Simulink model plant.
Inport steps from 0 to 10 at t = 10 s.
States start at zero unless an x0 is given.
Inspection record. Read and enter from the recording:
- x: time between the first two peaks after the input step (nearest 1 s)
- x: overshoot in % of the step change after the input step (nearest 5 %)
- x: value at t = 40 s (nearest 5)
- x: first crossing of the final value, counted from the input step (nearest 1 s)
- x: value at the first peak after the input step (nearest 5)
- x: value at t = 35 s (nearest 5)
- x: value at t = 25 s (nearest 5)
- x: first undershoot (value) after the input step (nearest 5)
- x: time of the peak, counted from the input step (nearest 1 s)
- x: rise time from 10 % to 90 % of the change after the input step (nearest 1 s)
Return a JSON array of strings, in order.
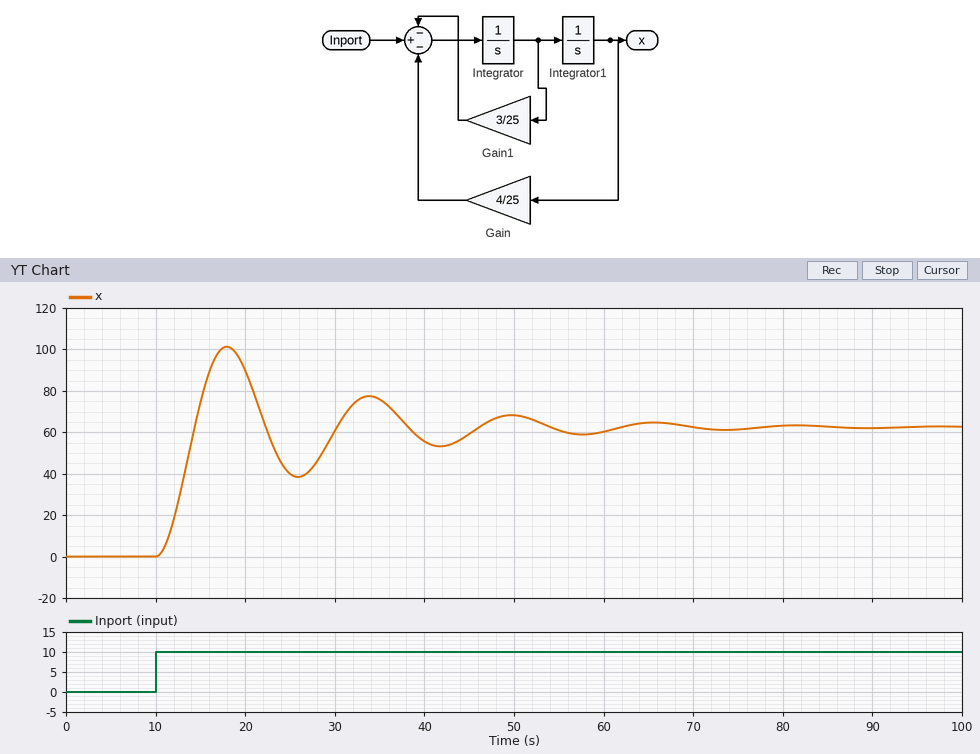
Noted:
["16 s", "60 %", "55", "4 s", "100", "75", "40", "40", "8 s", "3 s"]
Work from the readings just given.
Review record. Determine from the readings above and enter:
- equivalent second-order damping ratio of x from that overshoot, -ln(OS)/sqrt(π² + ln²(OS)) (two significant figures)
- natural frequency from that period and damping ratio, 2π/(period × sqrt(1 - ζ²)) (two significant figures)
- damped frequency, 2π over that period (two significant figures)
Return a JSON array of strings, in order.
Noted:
["0.16", "0.40 rad/s", "0.39 rad/s"]
